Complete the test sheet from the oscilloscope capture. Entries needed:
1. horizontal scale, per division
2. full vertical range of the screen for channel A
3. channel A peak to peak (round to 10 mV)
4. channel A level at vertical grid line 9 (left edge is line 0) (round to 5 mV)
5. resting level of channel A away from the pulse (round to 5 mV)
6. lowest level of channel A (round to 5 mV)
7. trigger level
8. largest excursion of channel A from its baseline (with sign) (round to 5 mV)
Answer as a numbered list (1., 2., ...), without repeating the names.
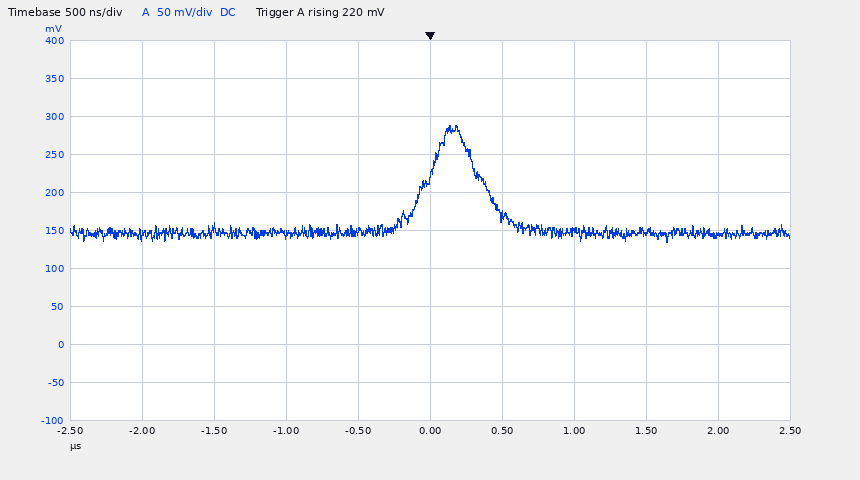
1. 500 ns
2. 500 mV
3. 150 mV
4. 145 mV
5. 145 mV
6. 135 mV
7. 220 mV
8. +140 mV
